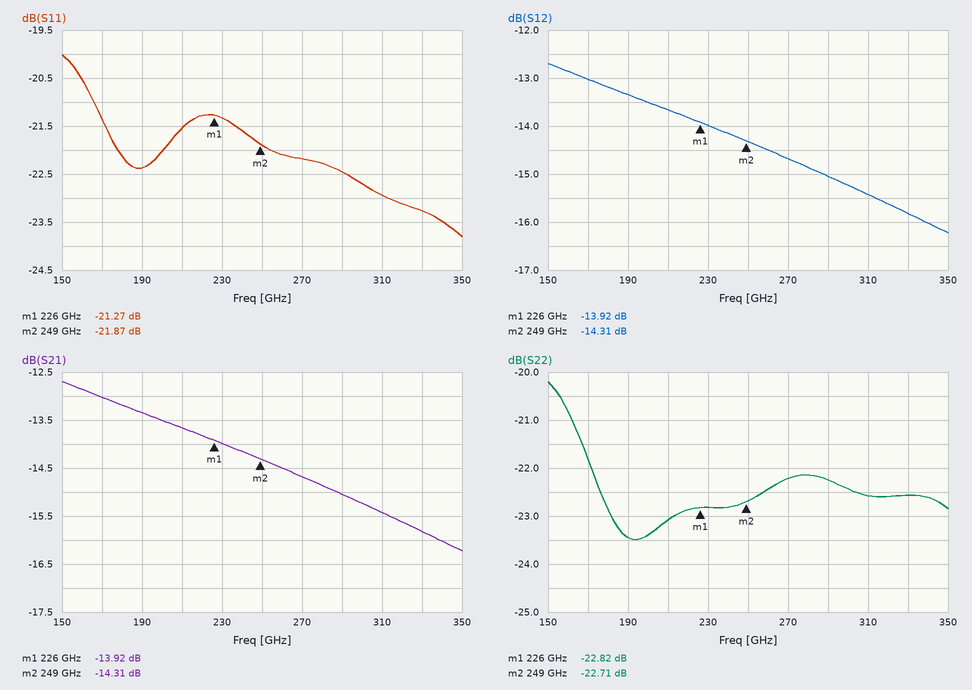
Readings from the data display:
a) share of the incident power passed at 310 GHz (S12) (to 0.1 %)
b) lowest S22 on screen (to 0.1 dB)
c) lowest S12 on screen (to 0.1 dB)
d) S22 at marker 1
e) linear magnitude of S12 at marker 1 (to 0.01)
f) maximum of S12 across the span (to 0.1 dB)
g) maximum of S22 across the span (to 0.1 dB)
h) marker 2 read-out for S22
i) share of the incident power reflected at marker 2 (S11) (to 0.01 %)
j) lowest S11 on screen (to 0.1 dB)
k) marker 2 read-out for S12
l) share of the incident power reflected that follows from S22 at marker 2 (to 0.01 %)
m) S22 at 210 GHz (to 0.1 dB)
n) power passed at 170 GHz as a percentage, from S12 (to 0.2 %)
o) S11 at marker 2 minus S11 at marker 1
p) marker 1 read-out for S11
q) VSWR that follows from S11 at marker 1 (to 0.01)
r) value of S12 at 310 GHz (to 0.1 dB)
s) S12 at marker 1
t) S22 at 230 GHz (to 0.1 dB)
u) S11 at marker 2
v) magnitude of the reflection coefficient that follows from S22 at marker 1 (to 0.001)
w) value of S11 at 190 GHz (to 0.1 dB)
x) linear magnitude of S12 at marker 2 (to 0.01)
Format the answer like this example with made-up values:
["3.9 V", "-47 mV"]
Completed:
["2.9 %", "-23.5 dB", "-16.2 dB", "-22.82 dB", "0.20", "-12.7 dB", "-20.2 dB", "-22.71 dB", "0.65 %", "-23.8 dB", "-14.31 dB", "0.54 %", "-23.1 dB", "5.0 %", "-0.60 dB", "-21.27 dB", "1.19", "-15.4 dB", "-13.92 dB", "-22.8 dB", "-21.87 dB", "0.072", "-22.4 dB", "0.19"]
